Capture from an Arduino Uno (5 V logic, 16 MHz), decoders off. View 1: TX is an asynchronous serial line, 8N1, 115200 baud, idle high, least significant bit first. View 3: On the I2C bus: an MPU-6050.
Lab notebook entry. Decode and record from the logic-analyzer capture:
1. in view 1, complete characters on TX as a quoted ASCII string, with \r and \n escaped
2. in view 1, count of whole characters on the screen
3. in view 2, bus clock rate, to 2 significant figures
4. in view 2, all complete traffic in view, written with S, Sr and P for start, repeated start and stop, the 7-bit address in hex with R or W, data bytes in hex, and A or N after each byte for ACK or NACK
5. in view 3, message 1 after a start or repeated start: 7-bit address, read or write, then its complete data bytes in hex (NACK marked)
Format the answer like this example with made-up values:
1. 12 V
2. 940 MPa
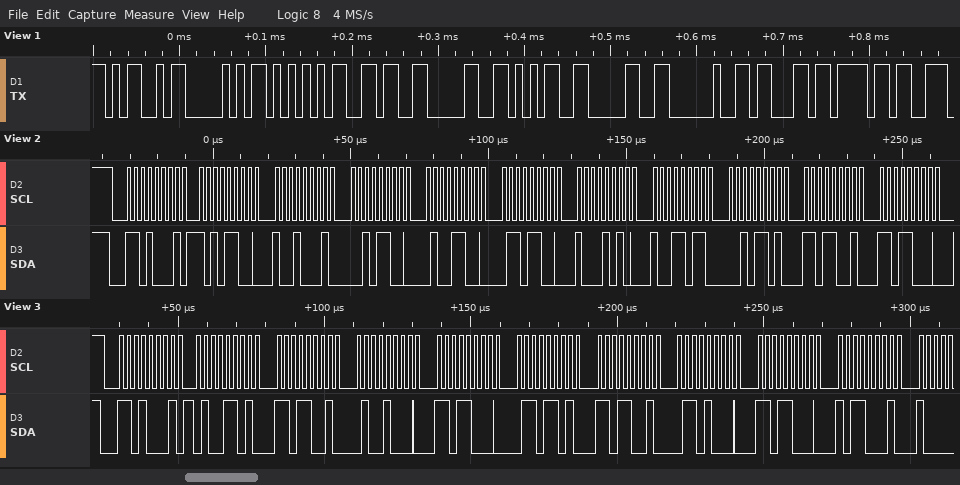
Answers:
1. "MPU6050 co"
2. 10
3. 400 kHz
4. S 68R A AC A 91 A 2C A 4C A 6C A 8A A 9B A 2D A D9 A D8 A
5. 0x68 read: 4D D9 48 D8 6D D9 68 D8 B1
